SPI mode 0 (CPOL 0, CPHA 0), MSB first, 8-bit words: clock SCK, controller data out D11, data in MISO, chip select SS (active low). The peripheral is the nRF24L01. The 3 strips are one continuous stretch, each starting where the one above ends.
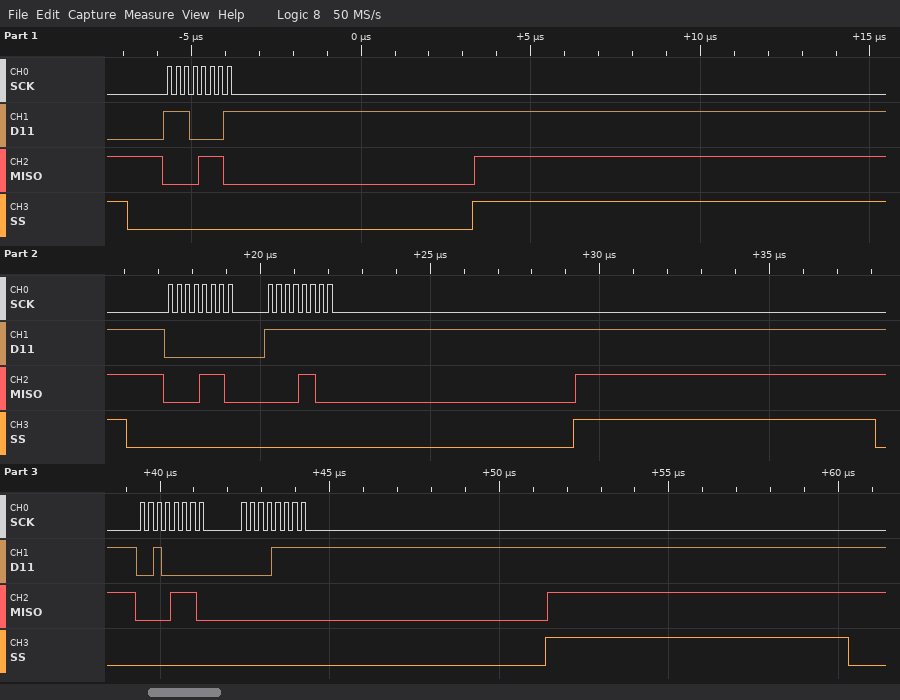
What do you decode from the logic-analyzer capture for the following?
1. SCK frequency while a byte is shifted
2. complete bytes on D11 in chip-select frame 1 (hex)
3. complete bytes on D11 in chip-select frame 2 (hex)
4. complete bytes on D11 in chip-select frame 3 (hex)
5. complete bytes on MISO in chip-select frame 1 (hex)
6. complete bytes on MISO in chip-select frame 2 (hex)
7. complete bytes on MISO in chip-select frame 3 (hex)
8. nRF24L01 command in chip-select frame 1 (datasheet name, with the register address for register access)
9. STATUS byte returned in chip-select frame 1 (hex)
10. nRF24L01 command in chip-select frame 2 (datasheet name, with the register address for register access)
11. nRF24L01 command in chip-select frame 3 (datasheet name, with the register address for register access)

4 MHz
E1
00 FF
20 0F
0E
0E 0C
0E 00
FLUSH_TX
0x0E
R_REGISTER 0x00
W_REGISTER 0x00
